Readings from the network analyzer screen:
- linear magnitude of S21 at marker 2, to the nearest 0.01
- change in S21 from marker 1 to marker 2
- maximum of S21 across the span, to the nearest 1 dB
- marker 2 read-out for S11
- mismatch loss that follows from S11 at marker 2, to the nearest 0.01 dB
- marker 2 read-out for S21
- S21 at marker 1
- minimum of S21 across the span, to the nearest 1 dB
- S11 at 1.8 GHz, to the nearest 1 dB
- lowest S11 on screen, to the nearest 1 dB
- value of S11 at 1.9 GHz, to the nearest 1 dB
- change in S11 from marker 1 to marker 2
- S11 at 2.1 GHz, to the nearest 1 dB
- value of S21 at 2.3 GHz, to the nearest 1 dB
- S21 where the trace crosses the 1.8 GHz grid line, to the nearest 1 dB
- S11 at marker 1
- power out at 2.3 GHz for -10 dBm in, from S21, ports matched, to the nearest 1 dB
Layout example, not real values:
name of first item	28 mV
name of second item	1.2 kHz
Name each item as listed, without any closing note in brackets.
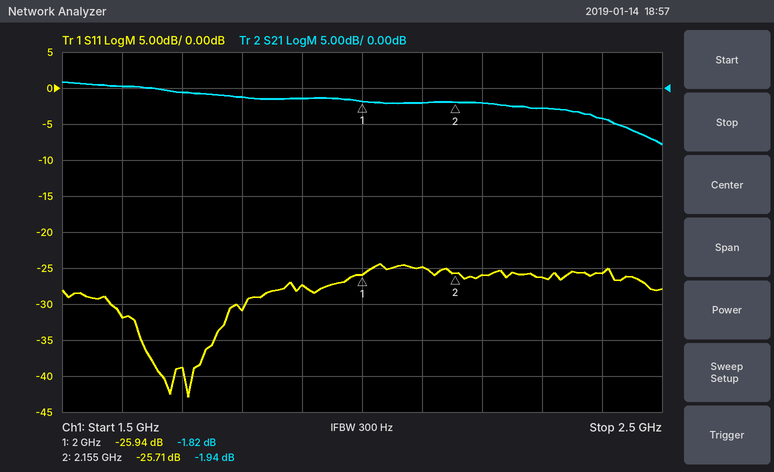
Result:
linear magnitude of S21 at marker 2, to the nearest 0.01	0.80
change in S21 from marker 1 to marker 2	-0.12 dB
maximum of S21 across the span, to the nearest 1 dB	1 dB
marker 2 read-out for S11	-25.71 dB
mismatch loss that follows from S11 at marker 2, to the nearest 0.01 dB	0.01 dB
marker 2 read-out for S21	-1.94 dB
S21 at marker 1	-1.82 dB
minimum of S21 across the span, to the nearest 1 dB	-8 dB
S11 at 1.8 GHz, to the nearest 1 dB	-31 dB
lowest S11 on screen, to the nearest 1 dB	-43 dB
value of S11 at 1.9 GHz, to the nearest 1 dB	-27 dB
change in S11 from marker 1 to marker 2	0.23 dB
S11 at 2.1 GHz, to the nearest 1 dB	-25 dB
value of S21 at 2.3 GHz, to the nearest 1 dB	-3 dB
S21 where the trace crosses the 1.8 GHz grid line, to the nearest 1 dB	-1 dB
S11 at marker 1	-25.94 dB
power out at 2.3 GHz for -10 dBm in, from S21, ports matched, to the nearest 1 dB	-13 dBm
